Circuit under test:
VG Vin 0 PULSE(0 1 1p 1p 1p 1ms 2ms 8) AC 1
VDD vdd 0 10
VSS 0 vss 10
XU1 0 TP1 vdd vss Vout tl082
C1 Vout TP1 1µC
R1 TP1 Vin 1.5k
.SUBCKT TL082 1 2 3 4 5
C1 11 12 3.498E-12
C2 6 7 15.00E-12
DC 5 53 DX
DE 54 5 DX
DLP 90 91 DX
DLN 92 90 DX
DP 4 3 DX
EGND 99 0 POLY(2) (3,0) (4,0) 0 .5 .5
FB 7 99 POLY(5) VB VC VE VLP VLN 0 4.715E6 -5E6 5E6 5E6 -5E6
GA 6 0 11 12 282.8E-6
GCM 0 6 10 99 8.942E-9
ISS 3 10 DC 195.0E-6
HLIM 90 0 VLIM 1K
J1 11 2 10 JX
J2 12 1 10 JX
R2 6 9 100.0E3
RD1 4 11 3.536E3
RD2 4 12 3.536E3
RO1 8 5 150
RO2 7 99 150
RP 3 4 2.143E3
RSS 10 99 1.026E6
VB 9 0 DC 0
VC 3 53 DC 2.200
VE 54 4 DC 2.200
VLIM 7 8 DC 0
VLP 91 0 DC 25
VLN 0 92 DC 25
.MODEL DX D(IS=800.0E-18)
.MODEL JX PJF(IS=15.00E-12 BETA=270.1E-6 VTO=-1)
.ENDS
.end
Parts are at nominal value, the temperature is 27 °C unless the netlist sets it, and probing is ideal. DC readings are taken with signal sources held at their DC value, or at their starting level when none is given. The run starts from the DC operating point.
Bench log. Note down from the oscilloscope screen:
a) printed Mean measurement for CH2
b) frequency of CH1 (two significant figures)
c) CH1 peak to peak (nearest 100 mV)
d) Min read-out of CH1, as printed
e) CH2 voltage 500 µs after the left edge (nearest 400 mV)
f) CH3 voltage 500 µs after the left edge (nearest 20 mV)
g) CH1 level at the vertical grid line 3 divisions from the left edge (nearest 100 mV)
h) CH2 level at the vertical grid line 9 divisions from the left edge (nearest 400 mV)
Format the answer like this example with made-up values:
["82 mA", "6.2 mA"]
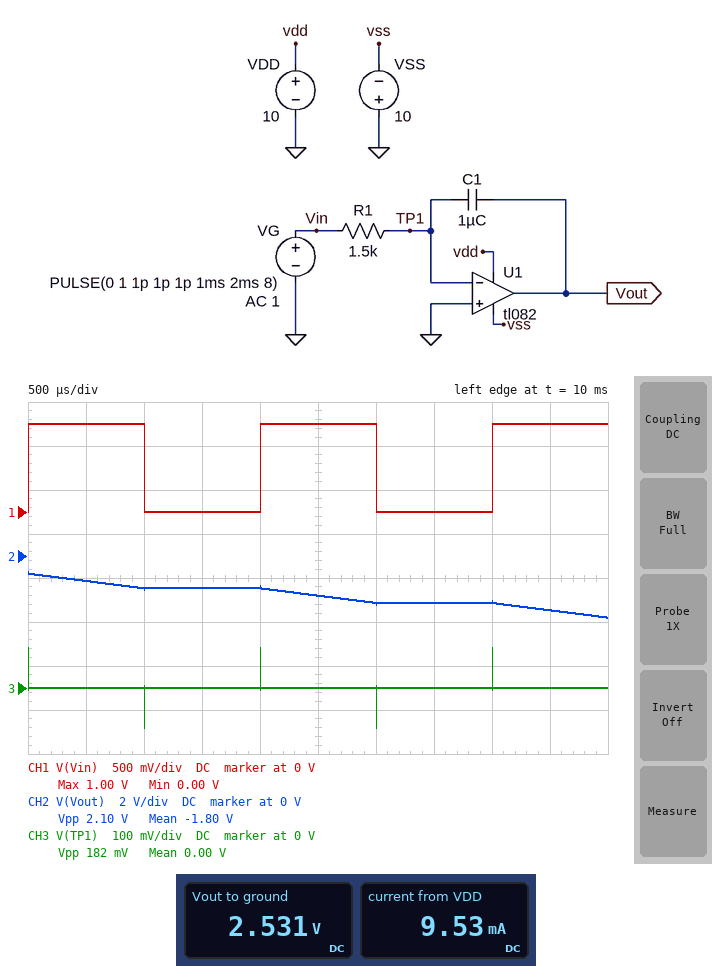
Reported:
["-1.80 V", "500 Hz", "1.0 V", "0.00 V", "-1.2 V", "0 V", "0 V", "-2.4 V"]
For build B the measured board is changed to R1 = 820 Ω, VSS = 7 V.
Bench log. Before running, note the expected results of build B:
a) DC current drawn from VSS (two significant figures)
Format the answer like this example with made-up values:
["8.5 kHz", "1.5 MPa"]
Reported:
["8.1 mA"]
